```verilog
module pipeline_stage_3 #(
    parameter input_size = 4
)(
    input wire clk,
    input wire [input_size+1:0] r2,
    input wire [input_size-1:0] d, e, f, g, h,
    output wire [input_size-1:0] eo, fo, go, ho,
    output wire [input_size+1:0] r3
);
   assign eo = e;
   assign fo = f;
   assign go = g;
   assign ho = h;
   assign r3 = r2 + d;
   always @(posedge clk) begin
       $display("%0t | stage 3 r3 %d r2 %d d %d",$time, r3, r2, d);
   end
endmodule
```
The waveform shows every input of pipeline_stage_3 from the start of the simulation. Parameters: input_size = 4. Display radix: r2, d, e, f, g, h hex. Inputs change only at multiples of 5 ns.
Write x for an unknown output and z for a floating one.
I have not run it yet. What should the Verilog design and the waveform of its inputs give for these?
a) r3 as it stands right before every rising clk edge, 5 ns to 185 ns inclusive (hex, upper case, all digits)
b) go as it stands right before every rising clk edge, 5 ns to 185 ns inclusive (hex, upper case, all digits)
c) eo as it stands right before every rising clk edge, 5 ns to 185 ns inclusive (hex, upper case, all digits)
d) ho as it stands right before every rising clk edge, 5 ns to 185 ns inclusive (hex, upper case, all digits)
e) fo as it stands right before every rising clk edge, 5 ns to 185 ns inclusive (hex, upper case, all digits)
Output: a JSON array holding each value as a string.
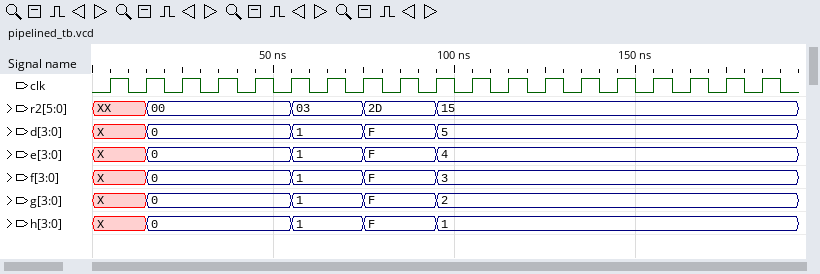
["x, x, 00, 00, 00, 00, 04, 04, 3C, 3C, 1A, 1A, 1A, 1A, 1A, 1A, 1A, 1A, 1A", "x, x, 0, 0, 0, 0, 1, 1, F, F, 2, 2, 2, 2, 2, 2, 2, 2, 2", "x, x, 0, 0, 0, 0, 1, 1, F, F, 4, 4, 4, 4, 4, 4, 4, 4, 4", "x, x, 0, 0, 0, 0, 1, 1, F, F, 1, 1, 1, 1, 1, 1, 1, 1, 1", "x, x, 0, 0, 0, 0, 1, 1, F, F, 3, 3, 3, 3, 3, 3, 3, 3, 3"]
